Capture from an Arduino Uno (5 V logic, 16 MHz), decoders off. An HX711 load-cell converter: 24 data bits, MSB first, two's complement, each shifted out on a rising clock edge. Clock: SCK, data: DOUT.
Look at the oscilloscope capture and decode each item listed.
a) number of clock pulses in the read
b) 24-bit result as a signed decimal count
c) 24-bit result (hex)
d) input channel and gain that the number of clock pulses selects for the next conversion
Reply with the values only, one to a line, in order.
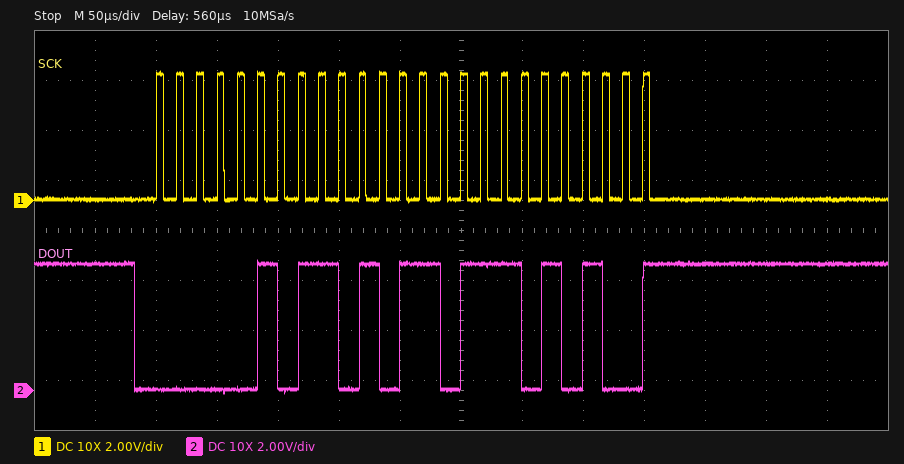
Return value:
25
372180
0x05ADD4
channel A, gain 128
